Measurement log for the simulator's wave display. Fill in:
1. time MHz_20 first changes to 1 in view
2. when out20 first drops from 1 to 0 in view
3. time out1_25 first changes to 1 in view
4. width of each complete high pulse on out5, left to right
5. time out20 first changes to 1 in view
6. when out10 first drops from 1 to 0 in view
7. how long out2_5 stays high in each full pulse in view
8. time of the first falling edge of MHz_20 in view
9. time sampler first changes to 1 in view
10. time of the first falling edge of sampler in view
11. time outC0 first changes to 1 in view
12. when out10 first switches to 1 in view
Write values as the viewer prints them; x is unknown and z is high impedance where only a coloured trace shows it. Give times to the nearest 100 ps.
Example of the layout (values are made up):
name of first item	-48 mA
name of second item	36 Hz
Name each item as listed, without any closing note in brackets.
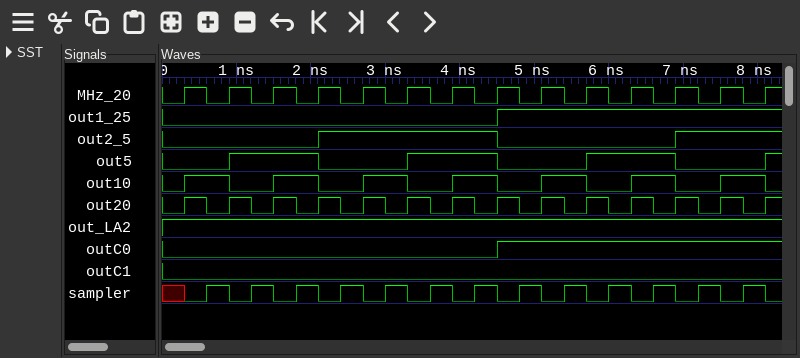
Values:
time MHz_20 first changes to 1 in view	300 ps
when out20 first drops from 1 to 0 in view	600 ps
time out1_25 first changes to 1 in view	4500 ps
width of each complete high pulse on out5, left to right	1200 ps, 1200 ps, 1200 ps
time out20 first changes to 1 in view	300 ps
when out10 first drops from 1 to 0 in view	900 ps
how long out2_5 stays high in each full pulse in view	2400 ps
time of the first falling edge of MHz_20 in view	600 ps
time sampler first changes to 1 in view	600 ps
time of the first falling edge of sampler in view	900 ps
time outC0 first changes to 1 in view	4500 ps
when out10 first switches to 1 in view	300 ps
